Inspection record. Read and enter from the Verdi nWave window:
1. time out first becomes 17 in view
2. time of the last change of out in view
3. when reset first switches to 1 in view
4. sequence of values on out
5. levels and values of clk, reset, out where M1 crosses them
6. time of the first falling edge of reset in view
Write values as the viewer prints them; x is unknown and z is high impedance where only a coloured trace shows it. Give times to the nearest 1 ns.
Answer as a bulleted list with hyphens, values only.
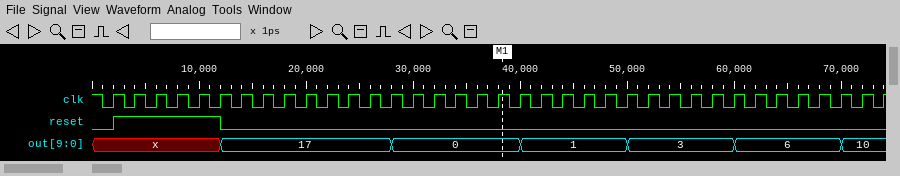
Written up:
- 12 ns
- 70 ns
- 2 ns
- x, 17, 0, 1, 3, 6, 10
- clk=1, reset=0, out=0
- 12 ns
